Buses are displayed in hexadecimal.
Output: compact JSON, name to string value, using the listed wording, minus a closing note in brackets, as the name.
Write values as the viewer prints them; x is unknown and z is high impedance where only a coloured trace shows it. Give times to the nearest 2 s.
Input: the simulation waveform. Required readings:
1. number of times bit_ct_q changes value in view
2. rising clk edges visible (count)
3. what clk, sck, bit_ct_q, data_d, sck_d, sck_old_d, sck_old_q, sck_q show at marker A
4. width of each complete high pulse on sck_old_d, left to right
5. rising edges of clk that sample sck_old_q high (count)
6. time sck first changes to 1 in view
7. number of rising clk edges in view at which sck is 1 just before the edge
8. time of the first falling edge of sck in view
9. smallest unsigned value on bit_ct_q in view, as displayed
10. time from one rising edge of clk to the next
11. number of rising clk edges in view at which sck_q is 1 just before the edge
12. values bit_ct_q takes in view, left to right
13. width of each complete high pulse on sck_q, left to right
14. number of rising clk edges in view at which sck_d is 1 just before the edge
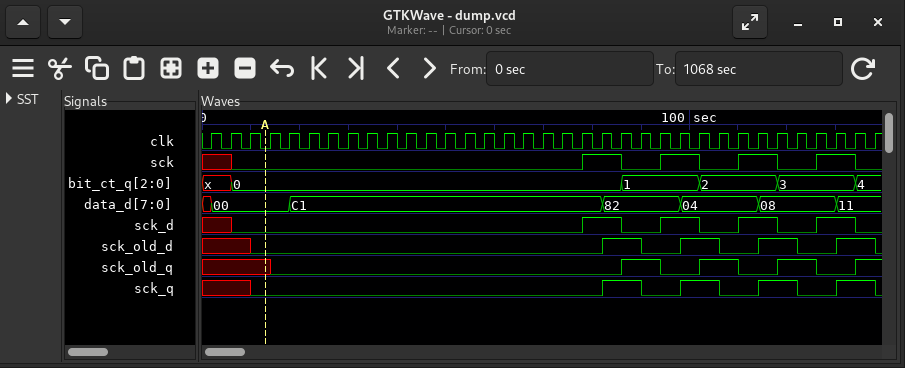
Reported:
{"number of times bit_ct_q changes value in view": "5", "rising clk edges visible": "35", "what clk, sck, bit_ct_q, data_d, sck_d, sck_old_d, sck_old_q, sck_q show at marker A": "clk=0, sck=0, bit_ct_q=0, data_d=00, sck_d=0, sck_old_d=0, sck_old_q=x, sck_q=0", "width of each complete high pulse on sck_old_d, left to right": "8 s, 8 s, 8 s, 8 s", "rising edges of clk that sample sck_old_q high": "7", "time sck first changes to 1 in view": "78 s", "number of rising clk edges in view at which sck is 1 just before the edge": "8", "time of the first falling edge of sck in view": "86 s", "smallest unsigned value on bit_ct_q in view, as displayed": "0", "time from one rising edge of clk to the next": "4 s", "number of rising clk edges in view at which sck_q is 1 just before the edge": "8", "values bit_ct_q takes in view, left to right": "x, 0, 1, 2, 3, 4", "width of each complete high pulse on sck_q, left to right": "8 s, 8 s, 8 s, 8 s", "number of rising clk edges in view at which sck_d is 1 just before the edge": "8"}
